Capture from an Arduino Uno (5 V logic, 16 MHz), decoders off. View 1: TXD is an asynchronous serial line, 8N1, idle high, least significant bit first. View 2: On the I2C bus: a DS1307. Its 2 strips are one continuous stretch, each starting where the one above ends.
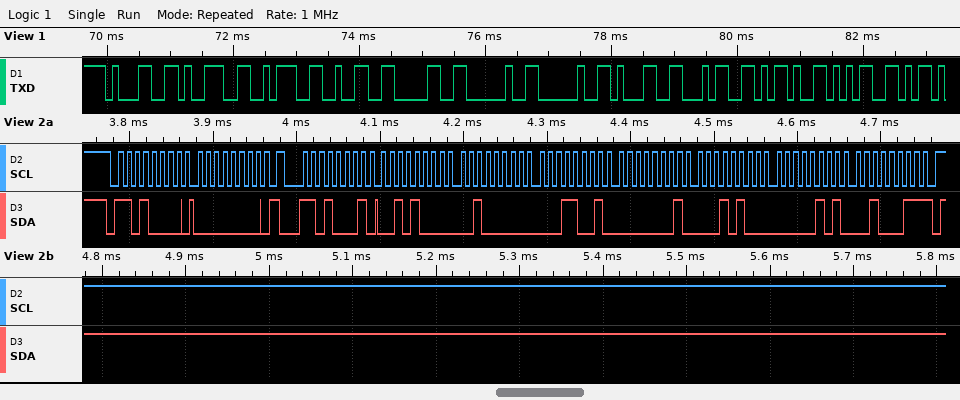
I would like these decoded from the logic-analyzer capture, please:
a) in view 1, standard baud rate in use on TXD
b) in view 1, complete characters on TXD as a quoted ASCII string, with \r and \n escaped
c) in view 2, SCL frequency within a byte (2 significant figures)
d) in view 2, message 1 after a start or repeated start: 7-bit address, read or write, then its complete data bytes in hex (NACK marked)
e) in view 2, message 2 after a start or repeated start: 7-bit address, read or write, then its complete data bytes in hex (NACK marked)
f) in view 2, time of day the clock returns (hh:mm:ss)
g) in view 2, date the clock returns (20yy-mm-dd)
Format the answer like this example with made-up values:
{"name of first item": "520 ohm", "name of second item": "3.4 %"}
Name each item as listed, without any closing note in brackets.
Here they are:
{"in view 1, standard baud rate in use on TXD": "9600 baud", "in view 1, complete characters on TXD as a quoted ASCII string, with \\r and \\n escaped": "\"19:20  14-5\"", "in view 2, SCL frequency within a byte": "100 kHz", "in view 2, message 1 after a start or repeated start: 7-bit address, read or write, then its complete data bytes in hex": "0x68 write: 00", "in view 2, message 2 after a start or repeated start: 7-bit address, read or write, then its complete data bytes in hex": "0x68 read: 28 20 19 01 14 05 23 NACK", "in view 2, time of day the clock returns": "19:20:28", "in view 2, date the clock returns": "2023-05-14"}
